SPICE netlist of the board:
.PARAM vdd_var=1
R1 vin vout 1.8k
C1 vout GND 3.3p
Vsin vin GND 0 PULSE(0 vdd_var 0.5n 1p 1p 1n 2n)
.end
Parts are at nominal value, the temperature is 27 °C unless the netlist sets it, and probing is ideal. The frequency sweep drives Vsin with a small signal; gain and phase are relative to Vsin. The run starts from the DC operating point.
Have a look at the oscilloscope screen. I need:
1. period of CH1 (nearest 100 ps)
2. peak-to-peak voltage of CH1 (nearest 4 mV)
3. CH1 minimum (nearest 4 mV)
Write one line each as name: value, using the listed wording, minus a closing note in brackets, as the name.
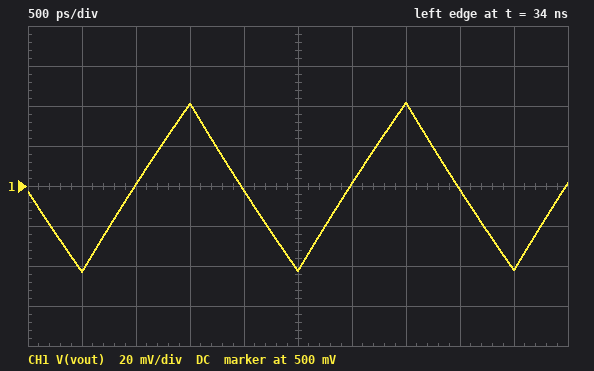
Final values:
period of CH1: 2.0 ns
peak-to-peak voltage of CH1: 84 mV
CH1 minimum: 456 mV
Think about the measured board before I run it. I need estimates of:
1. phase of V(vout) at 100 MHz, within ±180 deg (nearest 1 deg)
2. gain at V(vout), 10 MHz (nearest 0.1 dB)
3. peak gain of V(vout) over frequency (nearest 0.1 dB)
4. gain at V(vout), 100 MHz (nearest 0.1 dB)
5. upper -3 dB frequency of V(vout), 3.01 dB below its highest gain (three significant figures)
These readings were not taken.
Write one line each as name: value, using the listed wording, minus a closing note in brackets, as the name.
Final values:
phase of V(vout) at 100 MHz, within ±180 deg: -75 deg
gain at V(vout), 10 MHz: -0.6 dB
peak gain of V(vout) over frequency: 0 dB
gain at V(vout), 100 MHz: -11.7 dB
upper -3 dB frequency of V(vout), 3.01 dB below its highest gain: 26.8 MHz
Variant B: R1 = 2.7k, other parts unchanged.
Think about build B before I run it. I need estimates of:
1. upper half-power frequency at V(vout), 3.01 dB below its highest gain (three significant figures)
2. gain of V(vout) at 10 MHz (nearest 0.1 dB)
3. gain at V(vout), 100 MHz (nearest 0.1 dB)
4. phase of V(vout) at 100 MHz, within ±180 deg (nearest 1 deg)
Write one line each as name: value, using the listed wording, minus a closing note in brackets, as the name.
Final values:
upper half-power frequency at V(vout), 3.01 dB below its highest gain: 17.9 MHz
gain of V(vout) at 10 MHz: -1.2 dB
gain at V(vout), 100 MHz: -15.1 dB
phase of V(vout) at 100 MHz, within ±180 deg: -80 deg
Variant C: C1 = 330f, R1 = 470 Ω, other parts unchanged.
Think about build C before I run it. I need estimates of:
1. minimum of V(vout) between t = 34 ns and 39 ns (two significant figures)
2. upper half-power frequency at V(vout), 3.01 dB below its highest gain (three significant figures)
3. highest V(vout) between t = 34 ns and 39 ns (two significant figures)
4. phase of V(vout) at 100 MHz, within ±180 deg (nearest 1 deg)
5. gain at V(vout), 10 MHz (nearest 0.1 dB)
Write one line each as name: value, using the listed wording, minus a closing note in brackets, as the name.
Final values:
minimum of V(vout) between t = 34 ns and 39 ns: 1.6 mV
upper half-power frequency at V(vout), 3.01 dB below its highest gain: 1.03 GHz
highest V(vout) between t = 34 ns and 39 ns: 1.0 V
phase of V(vout) at 100 MHz, within ±180 deg: -6 deg
gain at V(vout), 10 MHz: 0 dB
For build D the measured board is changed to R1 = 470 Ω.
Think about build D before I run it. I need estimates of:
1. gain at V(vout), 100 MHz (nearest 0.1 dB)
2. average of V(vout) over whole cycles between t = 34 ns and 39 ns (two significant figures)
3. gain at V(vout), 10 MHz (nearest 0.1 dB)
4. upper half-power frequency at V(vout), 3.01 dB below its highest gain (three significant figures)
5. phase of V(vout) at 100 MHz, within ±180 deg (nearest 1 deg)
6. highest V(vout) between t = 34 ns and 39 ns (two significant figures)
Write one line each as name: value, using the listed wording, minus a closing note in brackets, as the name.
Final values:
gain at V(vout), 100 MHz: -2.9 dB
average of V(vout) over whole cycles between t = 34 ns and 39 ns: 500 mV
gain at V(vout), 10 MHz: 0 dB
upper half-power frequency at V(vout), 3.01 dB below its highest gain: 103 MHz
phase of V(vout) at 100 MHz, within ±180 deg: -44 deg
highest V(vout) between t = 34 ns and 39 ns: 660 mV
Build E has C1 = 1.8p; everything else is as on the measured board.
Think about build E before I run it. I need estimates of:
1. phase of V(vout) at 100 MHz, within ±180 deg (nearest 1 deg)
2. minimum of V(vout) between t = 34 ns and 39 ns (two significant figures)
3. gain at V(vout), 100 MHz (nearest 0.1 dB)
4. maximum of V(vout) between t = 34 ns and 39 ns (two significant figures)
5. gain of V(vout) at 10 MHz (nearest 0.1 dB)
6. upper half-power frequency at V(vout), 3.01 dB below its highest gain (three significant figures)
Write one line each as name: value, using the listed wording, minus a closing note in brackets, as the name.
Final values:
phase of V(vout) at 100 MHz, within ±180 deg: -64 deg
minimum of V(vout) between t = 34 ns and 39 ns: 420 mV
gain at V(vout), 100 MHz: -7.1 dB
maximum of V(vout) between t = 34 ns and 39 ns: 580 mV
gain of V(vout) at 10 MHz: -0.2 dB
upper half-power frequency at V(vout), 3.01 dB below its highest gain: 49.1 MHz
